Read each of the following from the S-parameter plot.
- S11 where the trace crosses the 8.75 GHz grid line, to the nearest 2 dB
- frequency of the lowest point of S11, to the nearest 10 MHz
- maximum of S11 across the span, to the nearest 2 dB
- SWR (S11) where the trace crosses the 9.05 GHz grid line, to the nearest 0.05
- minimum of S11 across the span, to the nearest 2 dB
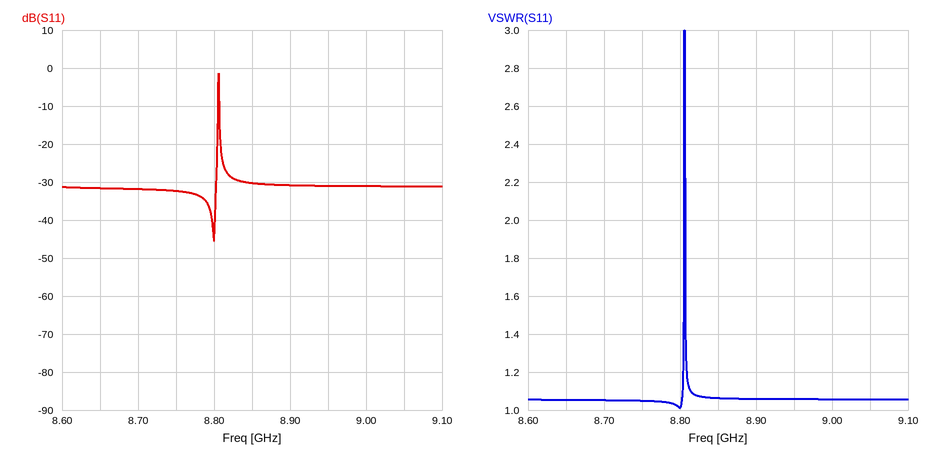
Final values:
-32 dB
8.80 GHz
-2 dB
1.05
-46 dB
